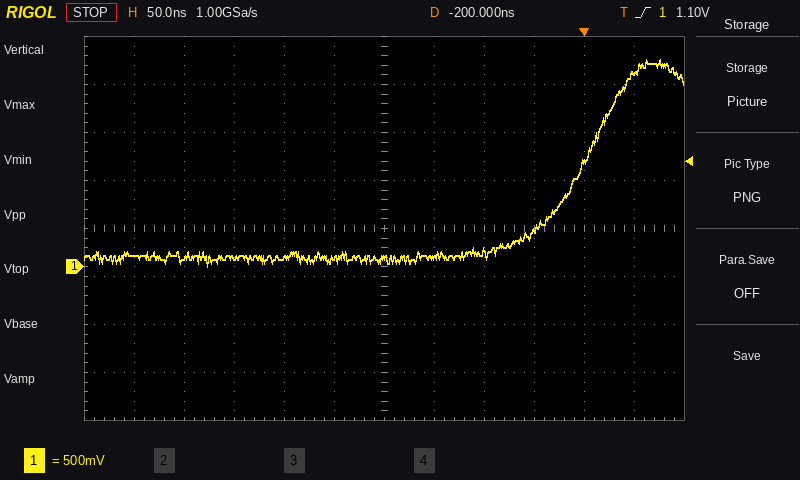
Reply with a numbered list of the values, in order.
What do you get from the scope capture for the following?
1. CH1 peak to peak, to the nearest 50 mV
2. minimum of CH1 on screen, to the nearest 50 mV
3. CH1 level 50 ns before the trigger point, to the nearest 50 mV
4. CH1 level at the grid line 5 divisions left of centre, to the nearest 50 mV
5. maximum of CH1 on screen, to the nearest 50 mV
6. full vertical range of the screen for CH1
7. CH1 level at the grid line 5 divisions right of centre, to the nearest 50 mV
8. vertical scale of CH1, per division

1. 2.15 V
2. 0 mV
3. 400 mV
4. 100 mV
5. 2.15 V
6. 4 V
7. 2.00 V
8. 500 mV
